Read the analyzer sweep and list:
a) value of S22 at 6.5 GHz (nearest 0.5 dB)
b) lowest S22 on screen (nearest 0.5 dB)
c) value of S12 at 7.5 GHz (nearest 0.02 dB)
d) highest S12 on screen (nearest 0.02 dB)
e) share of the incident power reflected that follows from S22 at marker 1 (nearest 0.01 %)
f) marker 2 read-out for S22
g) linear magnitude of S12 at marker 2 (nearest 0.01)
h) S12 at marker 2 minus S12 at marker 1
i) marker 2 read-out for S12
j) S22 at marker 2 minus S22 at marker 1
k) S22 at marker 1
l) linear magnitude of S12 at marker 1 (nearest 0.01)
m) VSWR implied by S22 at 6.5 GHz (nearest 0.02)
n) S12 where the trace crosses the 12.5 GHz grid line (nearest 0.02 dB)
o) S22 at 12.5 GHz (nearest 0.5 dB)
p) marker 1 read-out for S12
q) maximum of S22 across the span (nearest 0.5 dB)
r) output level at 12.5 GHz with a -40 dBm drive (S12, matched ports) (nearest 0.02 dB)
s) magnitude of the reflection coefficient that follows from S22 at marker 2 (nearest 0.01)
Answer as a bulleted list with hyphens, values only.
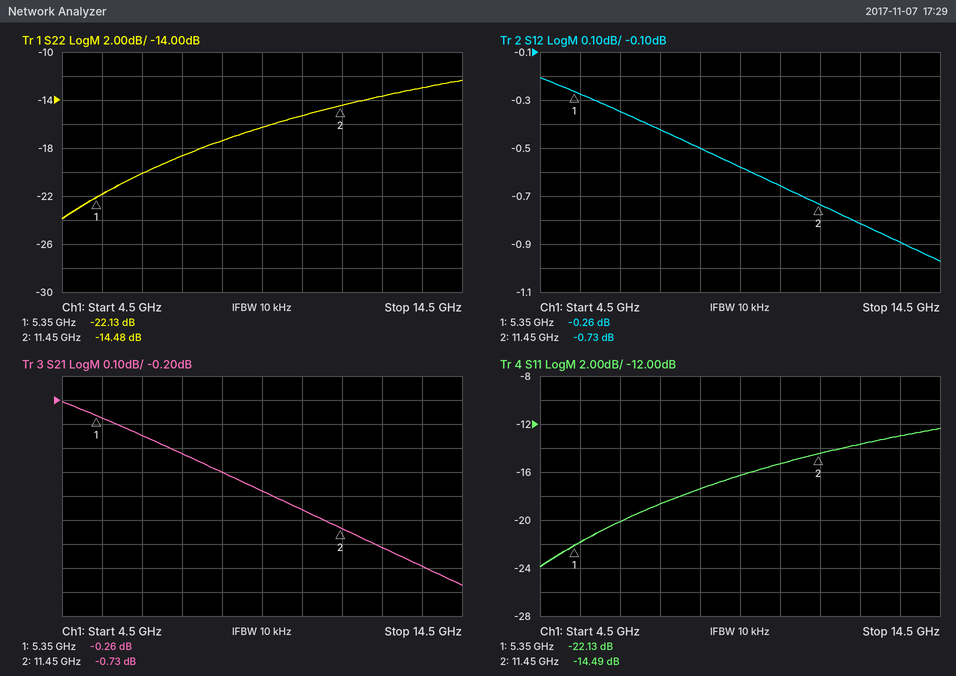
- -20.0 dB
- -24.0 dB
- -0.42 dB
- -0.20 dB
- 0.61 %
- -14.48 dB
- 0.92
- -0.47 dB
- -0.73 dB
- 7.65 dB
- -22.13 dB
- 0.97
- 1.22
- -0.82 dB
- -13.5 dB
- -0.26 dB
- -12.5 dB
- -40.82 dBm
- 0.19
